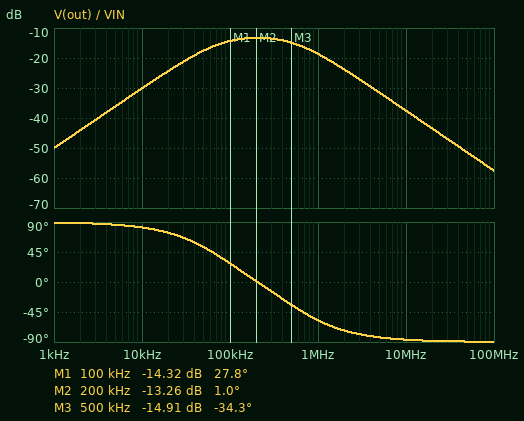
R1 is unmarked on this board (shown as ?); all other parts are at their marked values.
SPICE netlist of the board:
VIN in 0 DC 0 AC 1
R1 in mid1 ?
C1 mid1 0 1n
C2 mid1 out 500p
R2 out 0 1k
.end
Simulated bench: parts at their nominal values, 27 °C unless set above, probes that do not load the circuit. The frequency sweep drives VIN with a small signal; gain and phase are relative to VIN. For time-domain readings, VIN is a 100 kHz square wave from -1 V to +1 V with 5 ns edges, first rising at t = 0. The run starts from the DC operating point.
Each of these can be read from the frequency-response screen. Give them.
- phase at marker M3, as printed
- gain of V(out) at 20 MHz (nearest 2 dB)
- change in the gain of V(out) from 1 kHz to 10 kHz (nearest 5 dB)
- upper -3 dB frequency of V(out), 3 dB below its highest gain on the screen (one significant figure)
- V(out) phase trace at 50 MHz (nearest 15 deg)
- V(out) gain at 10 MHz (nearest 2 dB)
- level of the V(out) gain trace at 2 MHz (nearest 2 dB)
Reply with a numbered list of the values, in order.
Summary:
1. -34.3 deg
2. -44 dB
3. 20 dB
4. 700 kHz
5. -90 deg
6. -38 dB
7. -24 dB
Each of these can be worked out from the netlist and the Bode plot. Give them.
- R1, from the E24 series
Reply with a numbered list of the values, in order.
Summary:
1. 1.2 kΩ
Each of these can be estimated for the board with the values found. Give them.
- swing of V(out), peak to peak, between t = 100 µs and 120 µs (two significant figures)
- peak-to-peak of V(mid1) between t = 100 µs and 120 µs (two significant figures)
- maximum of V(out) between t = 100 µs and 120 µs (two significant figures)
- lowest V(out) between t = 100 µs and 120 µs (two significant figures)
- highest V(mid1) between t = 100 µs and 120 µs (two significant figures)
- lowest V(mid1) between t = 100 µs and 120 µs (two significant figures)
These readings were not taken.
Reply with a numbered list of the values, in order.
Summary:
1. 650 mV
2. 1.7 V
3. 330 mV
4. -330 mV
5. 870 mV
6. -870 mV
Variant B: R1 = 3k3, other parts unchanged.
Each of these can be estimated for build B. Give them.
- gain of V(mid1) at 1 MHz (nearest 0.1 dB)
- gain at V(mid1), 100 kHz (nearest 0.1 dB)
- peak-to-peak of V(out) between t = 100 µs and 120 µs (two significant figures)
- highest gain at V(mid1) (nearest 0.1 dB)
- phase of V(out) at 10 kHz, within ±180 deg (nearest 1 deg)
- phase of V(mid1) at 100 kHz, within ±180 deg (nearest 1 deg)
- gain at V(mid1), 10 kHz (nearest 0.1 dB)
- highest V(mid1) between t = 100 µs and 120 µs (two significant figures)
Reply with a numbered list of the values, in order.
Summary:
1. -26.9 dB
2. -10.3 dB
3. 230 mV
4. 0 dB
5. 71 deg
6. -67 deg
7. -0.4 dB
8. 470 mV
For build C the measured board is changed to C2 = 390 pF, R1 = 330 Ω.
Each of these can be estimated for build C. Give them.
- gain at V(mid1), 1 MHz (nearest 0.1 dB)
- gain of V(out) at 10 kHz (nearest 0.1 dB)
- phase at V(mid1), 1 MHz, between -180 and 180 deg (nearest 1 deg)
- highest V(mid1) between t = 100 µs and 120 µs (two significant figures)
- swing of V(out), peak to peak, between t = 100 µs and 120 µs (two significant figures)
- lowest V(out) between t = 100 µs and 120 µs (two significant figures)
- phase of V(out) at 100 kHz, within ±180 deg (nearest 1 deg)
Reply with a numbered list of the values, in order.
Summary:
1. -8.1 dB
2. -32.2 dB
3. -60 deg
4. 1.0 V
5. 1.4 V
6. -710 mV
7. 61 deg
